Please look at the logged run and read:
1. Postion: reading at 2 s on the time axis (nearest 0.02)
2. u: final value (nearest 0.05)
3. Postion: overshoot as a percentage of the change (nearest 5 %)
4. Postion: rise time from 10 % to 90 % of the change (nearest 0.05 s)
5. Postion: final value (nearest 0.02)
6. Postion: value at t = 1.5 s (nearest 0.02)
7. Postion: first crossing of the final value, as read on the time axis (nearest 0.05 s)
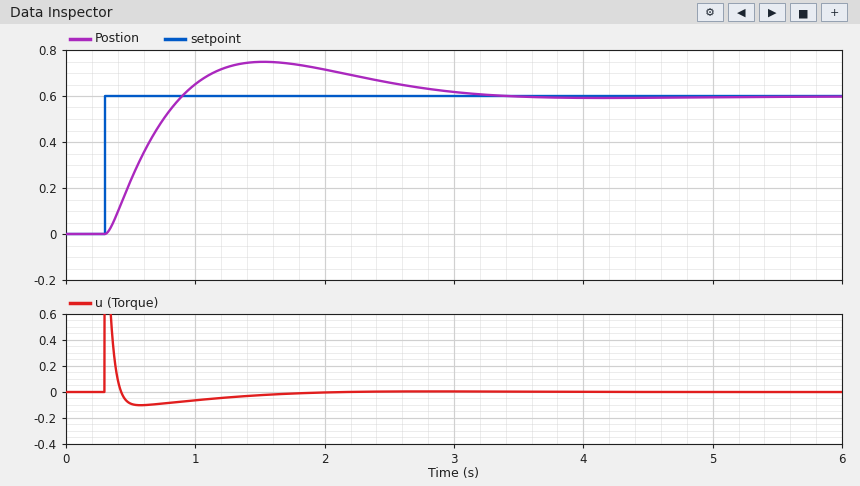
0.72
0.00
25 %
0.45 s
0.60
0.74
0.90 s
